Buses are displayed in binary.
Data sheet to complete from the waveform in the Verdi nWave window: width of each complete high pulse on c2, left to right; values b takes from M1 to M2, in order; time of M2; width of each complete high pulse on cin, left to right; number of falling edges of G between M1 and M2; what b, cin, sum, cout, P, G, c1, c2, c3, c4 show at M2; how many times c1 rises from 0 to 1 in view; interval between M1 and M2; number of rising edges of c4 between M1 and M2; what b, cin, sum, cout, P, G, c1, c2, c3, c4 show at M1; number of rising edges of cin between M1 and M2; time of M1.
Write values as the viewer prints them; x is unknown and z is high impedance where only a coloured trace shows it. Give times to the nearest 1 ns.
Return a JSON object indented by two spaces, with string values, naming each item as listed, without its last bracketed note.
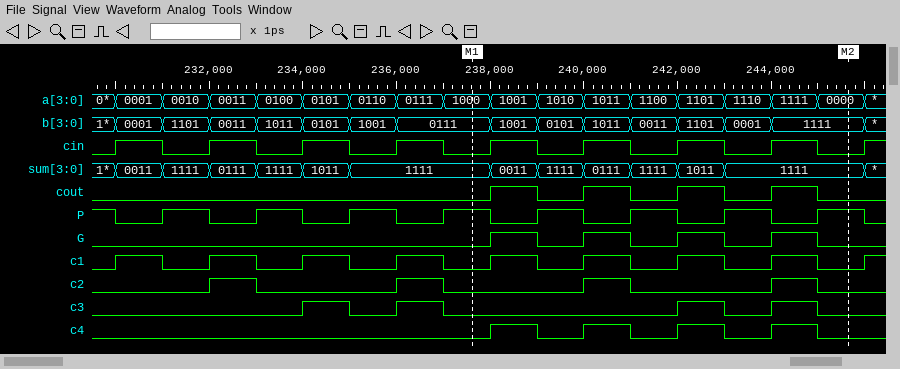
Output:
{
  "width of each complete high pulse on c2, left to right": "1 ns, 1 ns, 1 ns, 1 ns",
  "values b takes from M1 to M2, in order": "0111, 1001, 0101, 1011, 0011, 1101, 0001, 1111",
  "time of M2": "246 ns",
  "width of each complete high pulse on cin, left to right": "1 ns, 1 ns, 1 ns, 1 ns, 1 ns, 1 ns, 1 ns, 1 ns",
  "number of falling edges of G between M1 and M2": "4",
  "what b, cin, sum, cout, P, G, c1, c2, c3, c4 show at M2": "b=1111, cin=0, sum=1111, cout=0, P=1, G=0, c1=0, c2=0, c3=0, c4=0",
  "how many times c1 rises from 0 to 1 in view": "9",
  "interval between M1 and M2": "8 ns",
  "number of rising edges of c4 between M1 and M2": "4",
  "what b, cin, sum, cout, P, G, c1, c2, c3, c4 show at M1": "b=0111, cin=0, sum=1111, cout=0, P=1, G=0, c1=0, c2=0, c3=0, c4=0",
  "number of rising edges of cin between M1 and M2": "4",
  "time of M1": "238 ns"
}
